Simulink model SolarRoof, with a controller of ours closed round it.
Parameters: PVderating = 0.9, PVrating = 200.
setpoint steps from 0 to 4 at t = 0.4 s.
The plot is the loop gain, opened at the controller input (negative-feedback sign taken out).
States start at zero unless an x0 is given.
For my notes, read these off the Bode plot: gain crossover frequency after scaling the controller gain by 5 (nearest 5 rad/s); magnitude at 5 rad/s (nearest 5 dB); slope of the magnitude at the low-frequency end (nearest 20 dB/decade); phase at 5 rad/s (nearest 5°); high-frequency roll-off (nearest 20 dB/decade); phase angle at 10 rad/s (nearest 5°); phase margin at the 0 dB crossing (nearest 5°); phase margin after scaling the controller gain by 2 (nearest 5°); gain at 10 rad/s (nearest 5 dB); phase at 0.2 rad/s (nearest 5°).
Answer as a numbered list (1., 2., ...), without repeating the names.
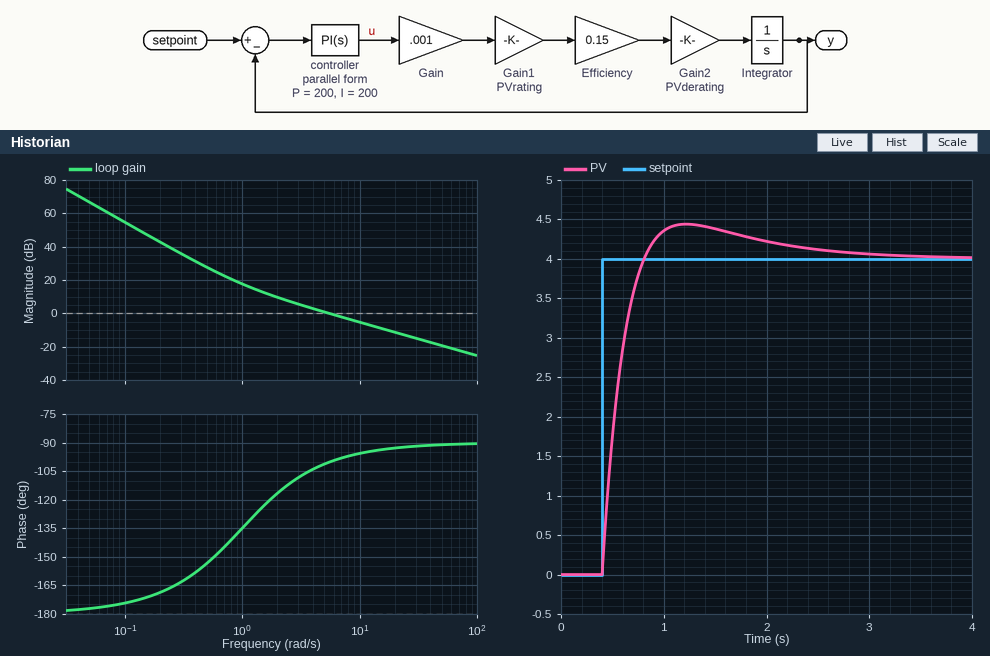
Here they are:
1. 25 rad/s
2. 0 dB
3. -40 dB/decade
4. -100°
5. -20 dB/decade
6. -95°
7. 80°
8. 85°
9. -5 dB
10. -170°
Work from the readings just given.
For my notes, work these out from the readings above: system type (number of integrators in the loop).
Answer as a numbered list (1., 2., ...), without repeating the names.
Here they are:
1. 2
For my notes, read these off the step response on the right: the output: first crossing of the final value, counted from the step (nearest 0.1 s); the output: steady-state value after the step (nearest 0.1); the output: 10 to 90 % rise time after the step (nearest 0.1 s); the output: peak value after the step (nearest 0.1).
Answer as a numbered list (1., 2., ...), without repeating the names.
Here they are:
1. 0.4 s
2. 4.0
3. 0.3 s
4. 4.4
